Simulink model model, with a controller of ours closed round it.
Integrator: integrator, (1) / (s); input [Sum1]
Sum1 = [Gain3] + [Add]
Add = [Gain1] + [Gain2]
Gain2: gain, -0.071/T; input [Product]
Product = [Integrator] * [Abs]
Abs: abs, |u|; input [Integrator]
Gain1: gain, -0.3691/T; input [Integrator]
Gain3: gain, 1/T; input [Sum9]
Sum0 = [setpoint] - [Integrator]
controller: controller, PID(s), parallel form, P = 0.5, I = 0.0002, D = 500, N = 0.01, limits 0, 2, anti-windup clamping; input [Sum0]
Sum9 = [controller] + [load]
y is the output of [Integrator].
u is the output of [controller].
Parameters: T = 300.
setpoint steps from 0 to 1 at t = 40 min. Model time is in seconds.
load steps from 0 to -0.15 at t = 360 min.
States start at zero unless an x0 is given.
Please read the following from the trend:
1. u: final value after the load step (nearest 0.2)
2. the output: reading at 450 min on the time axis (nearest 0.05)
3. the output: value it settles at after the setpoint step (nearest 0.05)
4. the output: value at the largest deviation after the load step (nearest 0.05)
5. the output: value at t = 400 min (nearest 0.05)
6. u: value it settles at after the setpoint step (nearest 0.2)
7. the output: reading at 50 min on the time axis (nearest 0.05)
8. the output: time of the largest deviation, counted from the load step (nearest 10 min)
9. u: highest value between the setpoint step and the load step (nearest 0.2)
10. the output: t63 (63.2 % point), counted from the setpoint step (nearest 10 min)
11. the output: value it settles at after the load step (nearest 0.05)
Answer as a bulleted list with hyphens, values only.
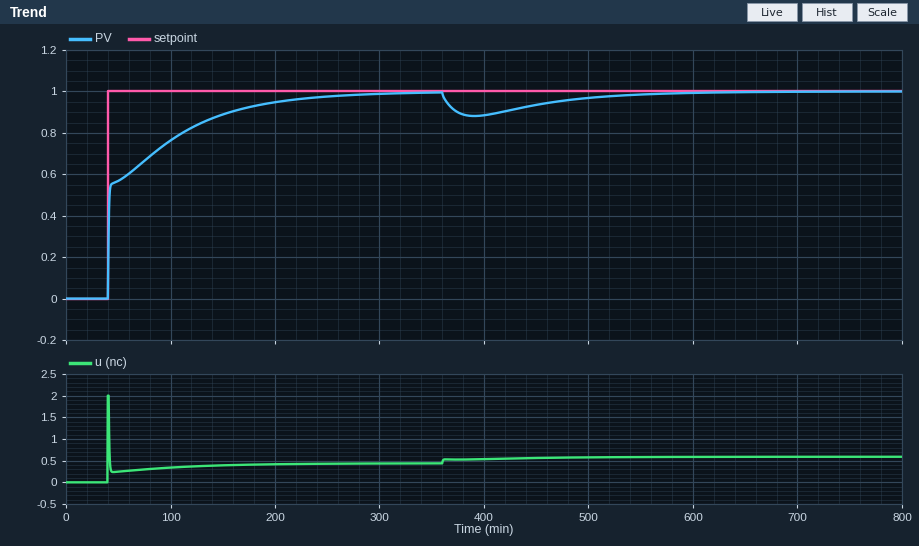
- 0.6
- 0.95
- 1.00
- 0.90
- 0.90
- 0.4
- 0.55
- 30 min
- 2.0
- 30 min
- 1.00
